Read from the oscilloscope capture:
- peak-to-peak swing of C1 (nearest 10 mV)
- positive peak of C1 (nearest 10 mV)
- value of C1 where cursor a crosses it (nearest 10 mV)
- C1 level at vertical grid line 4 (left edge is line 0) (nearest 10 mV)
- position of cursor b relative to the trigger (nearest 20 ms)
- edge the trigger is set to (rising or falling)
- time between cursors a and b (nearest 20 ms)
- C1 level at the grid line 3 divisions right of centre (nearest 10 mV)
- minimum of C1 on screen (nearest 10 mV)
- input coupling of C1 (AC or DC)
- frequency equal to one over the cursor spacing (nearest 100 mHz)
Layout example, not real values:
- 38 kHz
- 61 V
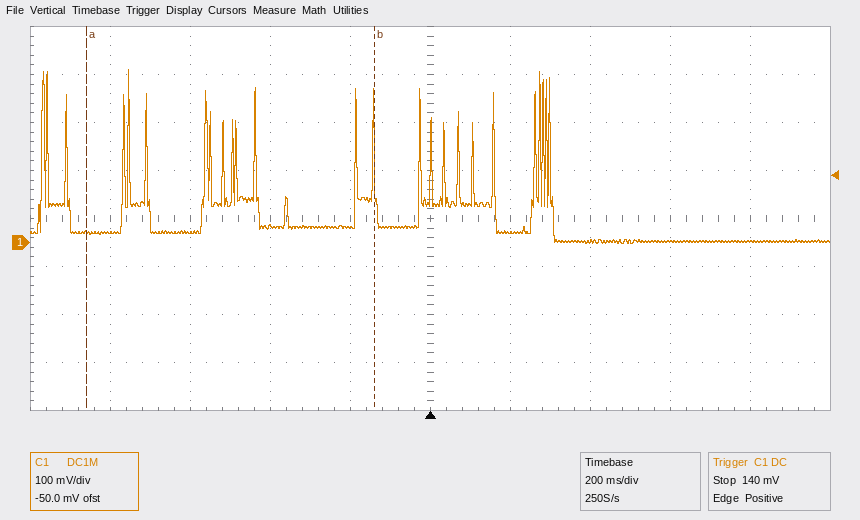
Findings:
- 360 mV
- 360 mV
- 20 mV
- 30 mV
- -140 ms
- rising
- 720 ms
- 0 mV
- 0 mV
- DC
- 1.4 Hz
